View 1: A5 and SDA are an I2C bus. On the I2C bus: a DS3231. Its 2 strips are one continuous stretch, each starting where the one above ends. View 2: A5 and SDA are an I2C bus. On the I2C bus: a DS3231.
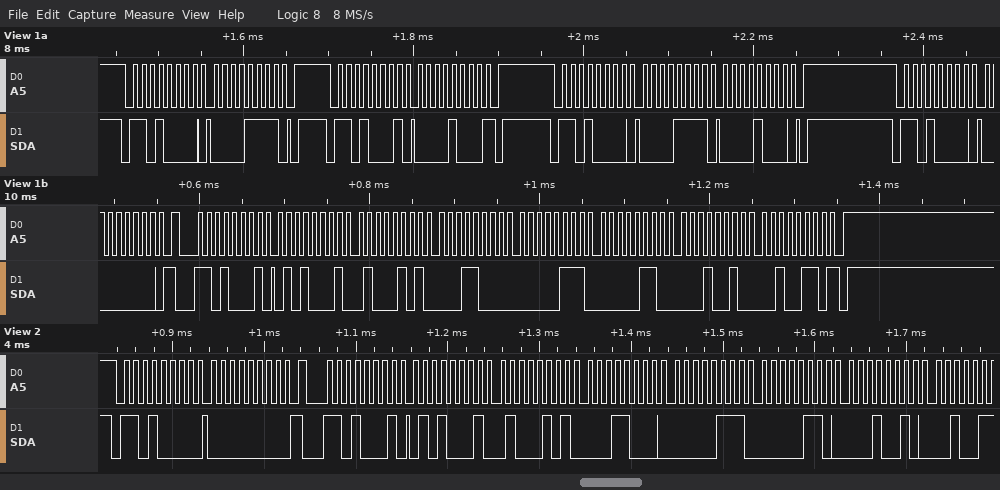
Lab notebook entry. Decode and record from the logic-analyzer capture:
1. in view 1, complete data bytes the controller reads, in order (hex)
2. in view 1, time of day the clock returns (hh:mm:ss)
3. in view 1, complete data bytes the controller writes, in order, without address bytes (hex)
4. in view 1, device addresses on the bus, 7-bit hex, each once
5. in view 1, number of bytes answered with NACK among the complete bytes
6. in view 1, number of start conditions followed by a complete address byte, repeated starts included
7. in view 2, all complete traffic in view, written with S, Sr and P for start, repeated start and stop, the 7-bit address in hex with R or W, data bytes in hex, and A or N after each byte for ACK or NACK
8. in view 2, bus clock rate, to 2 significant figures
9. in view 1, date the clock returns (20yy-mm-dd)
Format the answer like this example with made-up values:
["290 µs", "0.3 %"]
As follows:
["08 51 45 18 07 06 12 26", "18:45:51", "0F 0F 08 00", "0x68", "2", "5", "S 68W A 00 A Sr 68R A 51 A 45 A 18 A 07 A 06 A 12 A", "100 kHz", "2026-12-06"]
